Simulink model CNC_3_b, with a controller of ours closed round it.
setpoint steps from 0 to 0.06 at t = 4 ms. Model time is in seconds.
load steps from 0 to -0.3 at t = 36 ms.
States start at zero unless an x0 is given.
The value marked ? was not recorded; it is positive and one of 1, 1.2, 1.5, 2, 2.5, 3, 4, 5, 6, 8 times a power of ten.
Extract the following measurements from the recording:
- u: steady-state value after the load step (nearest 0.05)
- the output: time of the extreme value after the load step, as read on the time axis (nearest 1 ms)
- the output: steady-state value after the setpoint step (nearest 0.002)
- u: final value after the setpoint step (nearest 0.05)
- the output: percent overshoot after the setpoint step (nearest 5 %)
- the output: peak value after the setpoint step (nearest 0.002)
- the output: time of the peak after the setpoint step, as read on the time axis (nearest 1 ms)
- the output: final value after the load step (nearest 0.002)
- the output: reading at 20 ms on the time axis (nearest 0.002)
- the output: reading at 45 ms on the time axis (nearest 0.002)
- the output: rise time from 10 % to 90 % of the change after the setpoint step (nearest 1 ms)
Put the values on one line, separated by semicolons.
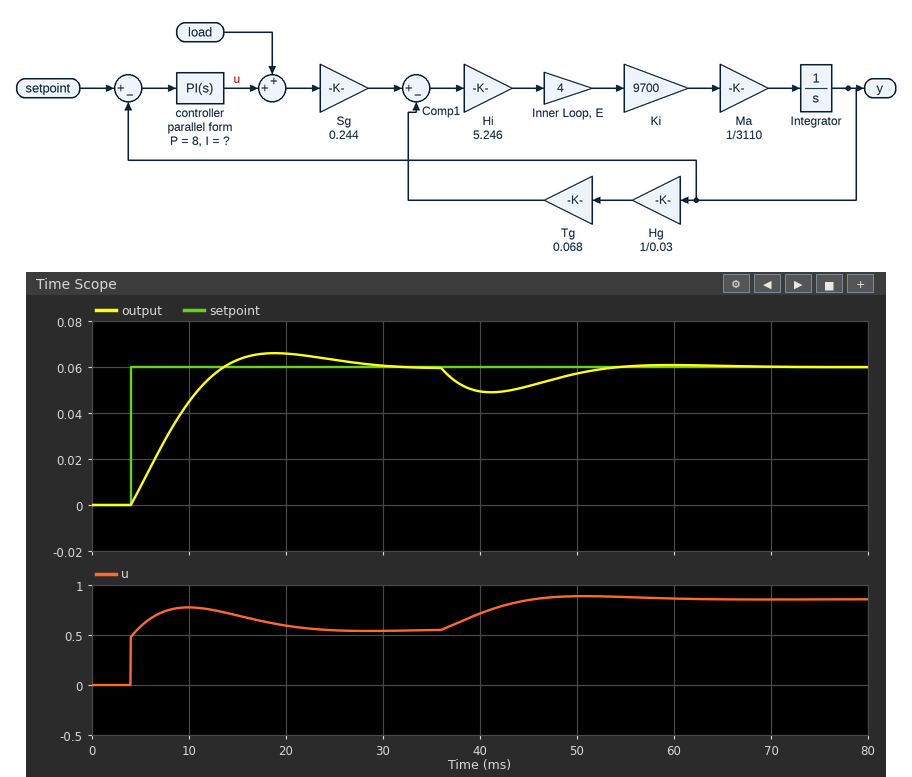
0.85; 41 ms; 0.060; 0.55; 10 %; 0.066; 19 ms; 0.060; 0.066; 0.052; 7 ms
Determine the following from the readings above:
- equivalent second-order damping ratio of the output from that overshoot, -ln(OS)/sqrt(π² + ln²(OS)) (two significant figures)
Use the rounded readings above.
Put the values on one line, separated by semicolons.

0.59
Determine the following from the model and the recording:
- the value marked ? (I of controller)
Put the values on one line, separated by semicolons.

3000
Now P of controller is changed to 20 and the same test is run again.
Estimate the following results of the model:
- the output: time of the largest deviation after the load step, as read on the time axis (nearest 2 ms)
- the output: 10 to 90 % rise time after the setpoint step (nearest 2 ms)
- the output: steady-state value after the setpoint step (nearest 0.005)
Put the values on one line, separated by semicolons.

40 ms; 6 ms; 0.060
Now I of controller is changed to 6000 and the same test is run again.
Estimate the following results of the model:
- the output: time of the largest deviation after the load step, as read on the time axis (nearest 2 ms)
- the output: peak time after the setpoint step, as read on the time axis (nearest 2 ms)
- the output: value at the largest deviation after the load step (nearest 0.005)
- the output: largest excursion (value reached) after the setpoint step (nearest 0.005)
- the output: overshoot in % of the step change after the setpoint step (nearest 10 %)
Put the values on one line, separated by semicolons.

40 ms; 14 ms; 0.050; 0.075; 20 %
